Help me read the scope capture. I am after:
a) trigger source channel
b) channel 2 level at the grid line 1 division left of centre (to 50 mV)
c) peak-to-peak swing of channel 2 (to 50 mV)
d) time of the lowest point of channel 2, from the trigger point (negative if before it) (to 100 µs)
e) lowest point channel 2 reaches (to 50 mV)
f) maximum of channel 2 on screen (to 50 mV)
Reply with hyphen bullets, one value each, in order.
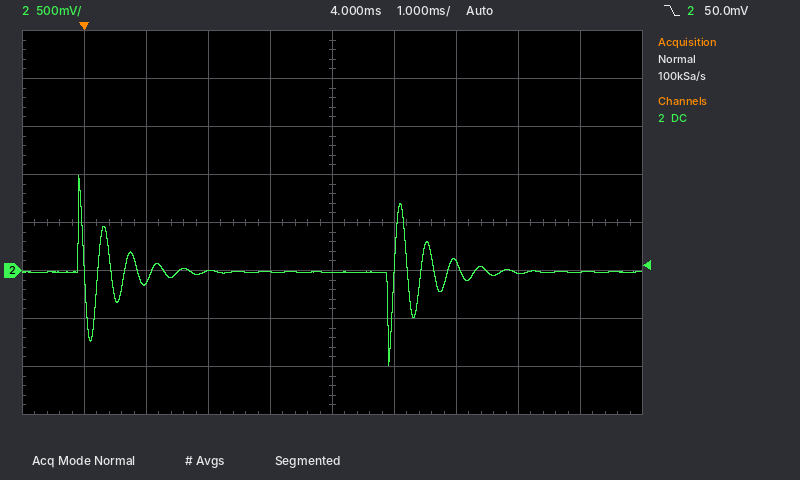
- channel 2
- 0 mV
- 2.00 V
- +4.9 ms
- -1.00 V
- 1.00 V
